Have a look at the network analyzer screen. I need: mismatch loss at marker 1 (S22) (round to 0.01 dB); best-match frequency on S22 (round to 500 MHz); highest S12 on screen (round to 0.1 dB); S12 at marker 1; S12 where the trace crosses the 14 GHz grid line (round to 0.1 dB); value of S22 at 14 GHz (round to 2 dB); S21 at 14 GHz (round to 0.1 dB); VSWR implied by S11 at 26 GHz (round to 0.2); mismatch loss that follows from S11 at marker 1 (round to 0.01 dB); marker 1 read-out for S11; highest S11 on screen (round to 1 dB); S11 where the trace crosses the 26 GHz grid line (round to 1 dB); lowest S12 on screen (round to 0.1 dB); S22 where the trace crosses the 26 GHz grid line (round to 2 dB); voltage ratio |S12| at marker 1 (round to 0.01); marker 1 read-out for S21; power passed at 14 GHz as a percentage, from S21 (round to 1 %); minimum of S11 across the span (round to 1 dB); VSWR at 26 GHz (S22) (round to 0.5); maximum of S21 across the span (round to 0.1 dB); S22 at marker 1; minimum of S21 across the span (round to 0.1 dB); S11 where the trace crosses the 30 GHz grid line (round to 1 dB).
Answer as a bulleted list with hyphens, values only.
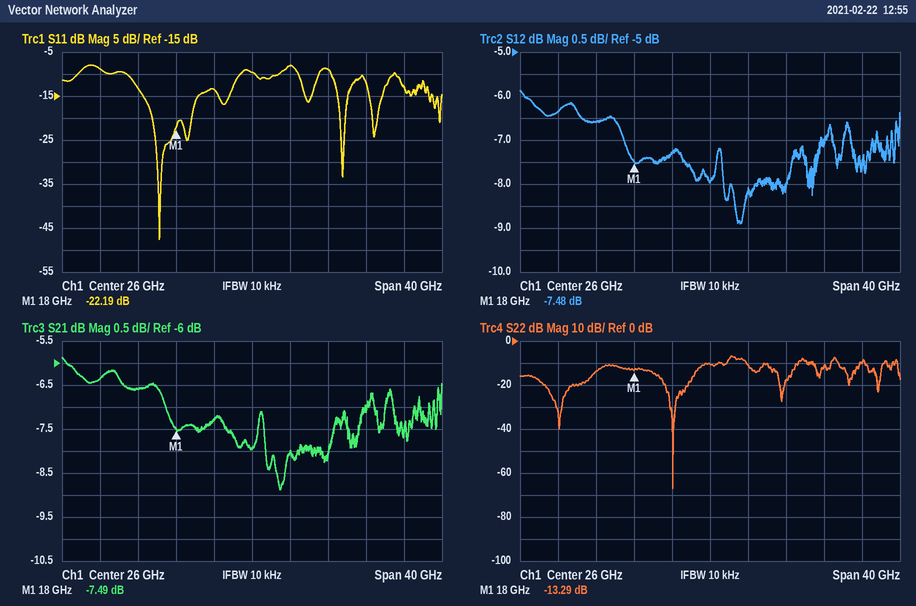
- 0.21 dB
- 22.0 GHz
- -5.9 dB
- -7.48 dB
- -6.6 dB
- -14 dB
- -6.6 dB
- 2.0
- 0.03 dB
- -22.19 dB
- -8 dB
- -10 dB
- -8.9 dB
- -10 dB
- 0.42
- -7.49 dB
- 22 %
- -48 dB
- 2.0
- -5.9 dB
- -13.29 dB
- -8.9 dB
- -8 dB
